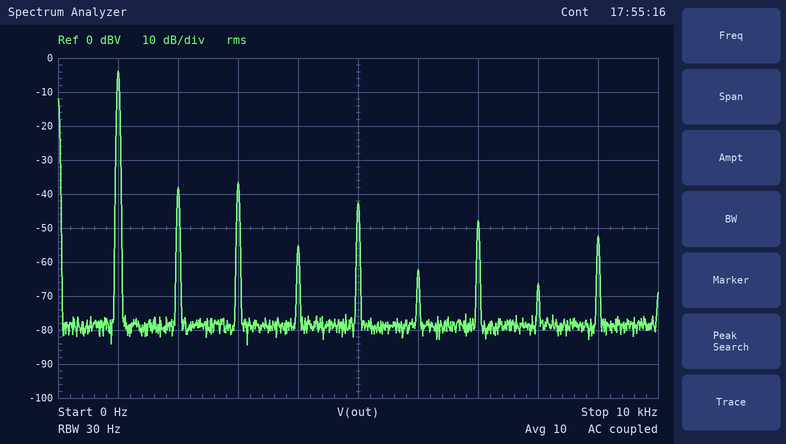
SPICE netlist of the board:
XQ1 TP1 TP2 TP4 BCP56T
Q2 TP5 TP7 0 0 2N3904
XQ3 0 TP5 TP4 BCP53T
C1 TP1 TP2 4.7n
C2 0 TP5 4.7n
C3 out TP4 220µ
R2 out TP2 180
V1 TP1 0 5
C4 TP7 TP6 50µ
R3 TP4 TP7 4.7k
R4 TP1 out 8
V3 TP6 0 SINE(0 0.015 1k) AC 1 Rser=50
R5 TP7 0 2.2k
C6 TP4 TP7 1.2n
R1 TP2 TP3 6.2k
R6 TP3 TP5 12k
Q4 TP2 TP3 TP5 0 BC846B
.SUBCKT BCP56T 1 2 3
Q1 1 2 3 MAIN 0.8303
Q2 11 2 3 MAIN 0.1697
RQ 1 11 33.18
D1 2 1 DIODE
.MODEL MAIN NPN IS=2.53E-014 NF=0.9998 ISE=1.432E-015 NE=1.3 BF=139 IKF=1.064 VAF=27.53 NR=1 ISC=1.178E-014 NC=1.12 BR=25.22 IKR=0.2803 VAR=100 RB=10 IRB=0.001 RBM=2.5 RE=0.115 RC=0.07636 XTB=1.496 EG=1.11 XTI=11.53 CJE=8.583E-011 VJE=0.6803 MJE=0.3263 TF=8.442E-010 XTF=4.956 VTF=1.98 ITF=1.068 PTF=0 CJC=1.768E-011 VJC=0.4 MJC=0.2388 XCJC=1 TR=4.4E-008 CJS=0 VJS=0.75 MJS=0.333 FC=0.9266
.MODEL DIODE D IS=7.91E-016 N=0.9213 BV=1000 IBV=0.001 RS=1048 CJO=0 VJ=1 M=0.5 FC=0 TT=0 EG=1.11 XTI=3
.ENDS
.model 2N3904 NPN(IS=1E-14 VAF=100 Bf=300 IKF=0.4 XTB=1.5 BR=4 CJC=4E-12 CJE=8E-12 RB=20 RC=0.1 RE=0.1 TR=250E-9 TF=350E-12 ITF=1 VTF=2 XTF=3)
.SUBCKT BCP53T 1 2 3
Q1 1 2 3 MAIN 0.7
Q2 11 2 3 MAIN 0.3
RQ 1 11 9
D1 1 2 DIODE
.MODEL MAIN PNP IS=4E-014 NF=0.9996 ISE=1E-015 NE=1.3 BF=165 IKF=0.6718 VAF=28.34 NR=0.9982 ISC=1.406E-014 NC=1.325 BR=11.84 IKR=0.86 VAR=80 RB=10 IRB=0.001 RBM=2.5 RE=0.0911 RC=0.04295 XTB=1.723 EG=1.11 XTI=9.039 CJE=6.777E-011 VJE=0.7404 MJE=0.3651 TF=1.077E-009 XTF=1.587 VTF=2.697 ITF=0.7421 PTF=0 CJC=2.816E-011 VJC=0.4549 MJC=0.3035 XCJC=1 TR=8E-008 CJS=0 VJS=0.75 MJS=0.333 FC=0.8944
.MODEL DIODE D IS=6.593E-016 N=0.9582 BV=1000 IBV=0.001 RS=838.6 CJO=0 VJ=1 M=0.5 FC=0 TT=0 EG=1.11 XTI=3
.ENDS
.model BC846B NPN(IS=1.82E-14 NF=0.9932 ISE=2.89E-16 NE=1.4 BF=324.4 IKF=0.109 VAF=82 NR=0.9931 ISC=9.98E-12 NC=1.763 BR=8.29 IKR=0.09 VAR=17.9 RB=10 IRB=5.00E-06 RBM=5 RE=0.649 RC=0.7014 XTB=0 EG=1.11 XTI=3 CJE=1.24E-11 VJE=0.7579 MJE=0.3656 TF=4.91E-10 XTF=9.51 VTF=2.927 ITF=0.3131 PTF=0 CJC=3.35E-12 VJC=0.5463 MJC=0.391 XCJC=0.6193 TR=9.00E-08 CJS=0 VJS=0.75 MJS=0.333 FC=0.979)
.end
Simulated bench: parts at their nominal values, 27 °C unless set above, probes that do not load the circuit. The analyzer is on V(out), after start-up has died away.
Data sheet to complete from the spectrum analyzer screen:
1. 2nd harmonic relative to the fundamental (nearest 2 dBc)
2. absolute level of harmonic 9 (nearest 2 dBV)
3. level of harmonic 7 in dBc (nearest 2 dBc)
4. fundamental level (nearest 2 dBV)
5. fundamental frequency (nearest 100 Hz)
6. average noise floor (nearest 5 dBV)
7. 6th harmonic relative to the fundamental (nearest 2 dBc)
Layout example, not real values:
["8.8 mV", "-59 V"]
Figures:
["-34 dBc", "-52 dBV", "-44 dBc", "-4 dBV", "1.0 kHz", "-80 dBV", "-58 dBc"]
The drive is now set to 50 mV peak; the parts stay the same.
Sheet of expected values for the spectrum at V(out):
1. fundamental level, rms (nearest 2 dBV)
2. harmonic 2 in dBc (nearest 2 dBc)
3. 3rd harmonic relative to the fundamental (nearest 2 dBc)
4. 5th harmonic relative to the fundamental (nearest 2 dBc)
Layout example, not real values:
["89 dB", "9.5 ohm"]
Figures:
["4 dBV", "-28 dBc", "-16 dBc", "-36 dBc"]
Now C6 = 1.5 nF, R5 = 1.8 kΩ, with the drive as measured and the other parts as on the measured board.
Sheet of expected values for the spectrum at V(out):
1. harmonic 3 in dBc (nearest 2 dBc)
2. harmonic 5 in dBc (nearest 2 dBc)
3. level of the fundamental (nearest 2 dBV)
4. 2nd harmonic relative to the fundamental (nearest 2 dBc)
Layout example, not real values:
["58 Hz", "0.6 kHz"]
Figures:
["-28 dBc", "-34 dBc", "-4 dBV", "-32 dBc"]
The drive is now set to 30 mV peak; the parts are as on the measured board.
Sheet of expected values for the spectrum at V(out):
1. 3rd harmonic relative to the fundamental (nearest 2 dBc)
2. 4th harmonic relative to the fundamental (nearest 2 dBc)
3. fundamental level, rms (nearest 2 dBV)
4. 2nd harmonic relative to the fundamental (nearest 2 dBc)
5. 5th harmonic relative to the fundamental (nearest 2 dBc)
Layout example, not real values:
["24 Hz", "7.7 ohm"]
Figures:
["-26 dBc", "-34 dBc", "2 dBV", "-38 dBc", "-30 dBc"]
